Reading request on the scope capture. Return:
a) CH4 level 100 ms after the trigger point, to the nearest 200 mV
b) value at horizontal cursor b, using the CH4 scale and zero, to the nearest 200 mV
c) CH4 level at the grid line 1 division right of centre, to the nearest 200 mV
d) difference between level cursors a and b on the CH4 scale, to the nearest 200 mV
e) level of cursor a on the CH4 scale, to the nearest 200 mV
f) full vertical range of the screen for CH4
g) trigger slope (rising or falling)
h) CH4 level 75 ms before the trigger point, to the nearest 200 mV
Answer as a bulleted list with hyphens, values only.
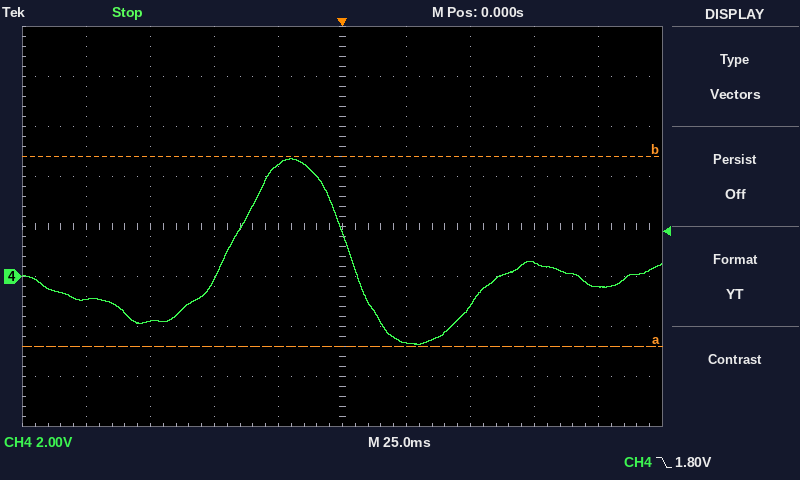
- -400 mV
- 4.8 V
- -2.6 V
- 7.6 V
- -2.8 V
- 16 V
- falling
- -1.8 V
